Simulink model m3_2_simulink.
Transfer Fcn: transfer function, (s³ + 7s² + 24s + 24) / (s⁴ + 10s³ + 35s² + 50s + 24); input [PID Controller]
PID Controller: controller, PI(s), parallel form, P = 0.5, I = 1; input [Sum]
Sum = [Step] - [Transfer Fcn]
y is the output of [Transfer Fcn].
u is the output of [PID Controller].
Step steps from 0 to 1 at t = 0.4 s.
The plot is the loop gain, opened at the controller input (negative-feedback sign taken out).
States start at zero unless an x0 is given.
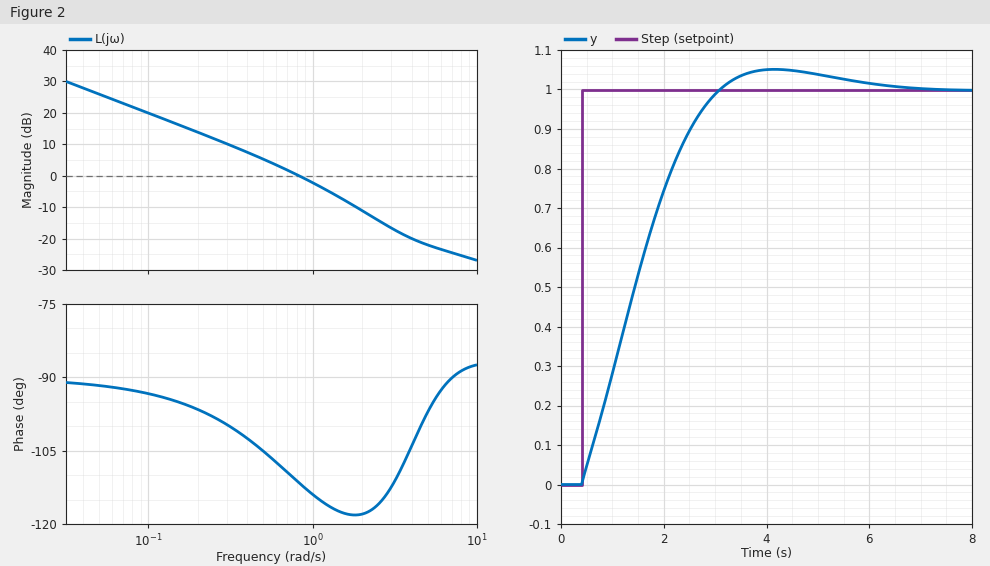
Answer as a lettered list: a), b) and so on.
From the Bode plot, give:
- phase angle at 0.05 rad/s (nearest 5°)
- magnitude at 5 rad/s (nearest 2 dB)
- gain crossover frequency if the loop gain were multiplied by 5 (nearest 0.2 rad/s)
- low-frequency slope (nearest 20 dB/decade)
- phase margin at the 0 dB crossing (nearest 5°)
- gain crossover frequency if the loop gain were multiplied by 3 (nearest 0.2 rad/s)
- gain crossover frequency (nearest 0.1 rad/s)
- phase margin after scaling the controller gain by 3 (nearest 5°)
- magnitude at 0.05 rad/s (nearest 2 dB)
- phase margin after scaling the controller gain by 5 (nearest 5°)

a) -90°
b) -22 dB
c) 2.4 rad/s
d) -20 dB/decade
e) 70°
f) 1.8 rad/s
g) 0.8 rad/s
h) 60°
i) 26 dB
j) 65°
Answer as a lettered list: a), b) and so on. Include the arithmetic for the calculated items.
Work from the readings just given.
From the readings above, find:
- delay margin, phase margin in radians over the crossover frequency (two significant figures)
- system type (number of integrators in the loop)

a) 70 × π / 180 / 0.8 = 1.5 s
b) 1
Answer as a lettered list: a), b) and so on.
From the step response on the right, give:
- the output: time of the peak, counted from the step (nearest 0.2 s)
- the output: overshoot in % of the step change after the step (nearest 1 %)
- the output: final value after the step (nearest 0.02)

a) 3.8 s
b) 5 %
c) 1.00
